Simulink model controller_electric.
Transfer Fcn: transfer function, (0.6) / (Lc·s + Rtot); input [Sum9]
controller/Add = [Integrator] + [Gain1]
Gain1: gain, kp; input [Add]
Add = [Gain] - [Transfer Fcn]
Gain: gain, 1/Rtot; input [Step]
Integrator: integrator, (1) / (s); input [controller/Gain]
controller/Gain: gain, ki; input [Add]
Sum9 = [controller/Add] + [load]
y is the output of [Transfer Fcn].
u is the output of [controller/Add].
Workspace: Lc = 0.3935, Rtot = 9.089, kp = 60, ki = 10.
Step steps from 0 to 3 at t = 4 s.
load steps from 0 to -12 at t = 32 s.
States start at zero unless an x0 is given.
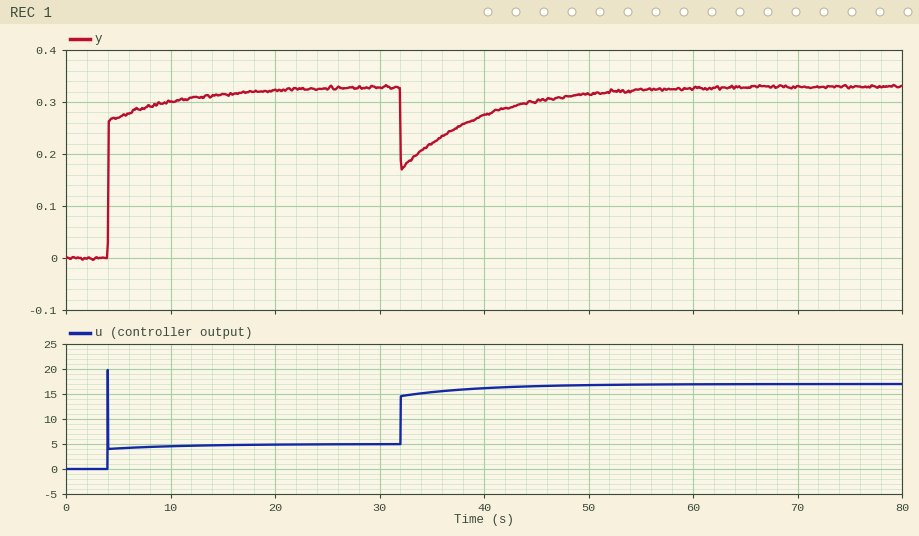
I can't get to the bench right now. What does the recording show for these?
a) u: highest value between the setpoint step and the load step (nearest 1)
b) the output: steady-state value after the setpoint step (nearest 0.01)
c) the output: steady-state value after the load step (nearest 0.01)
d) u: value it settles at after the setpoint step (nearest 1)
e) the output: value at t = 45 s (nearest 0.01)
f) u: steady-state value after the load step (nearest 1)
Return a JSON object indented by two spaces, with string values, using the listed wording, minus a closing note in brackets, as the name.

{
  "u: highest value between the setpoint step and the load step": "20",
  "the output: steady-state value after the setpoint step": "0.33",
  "the output: steady-state value after the load step": "0.33",
  "u: value it settles at after the setpoint step": "5",
  "the output: value at t = 45 s": "0.30",
  "u: steady-state value after the load step": "17"
}
